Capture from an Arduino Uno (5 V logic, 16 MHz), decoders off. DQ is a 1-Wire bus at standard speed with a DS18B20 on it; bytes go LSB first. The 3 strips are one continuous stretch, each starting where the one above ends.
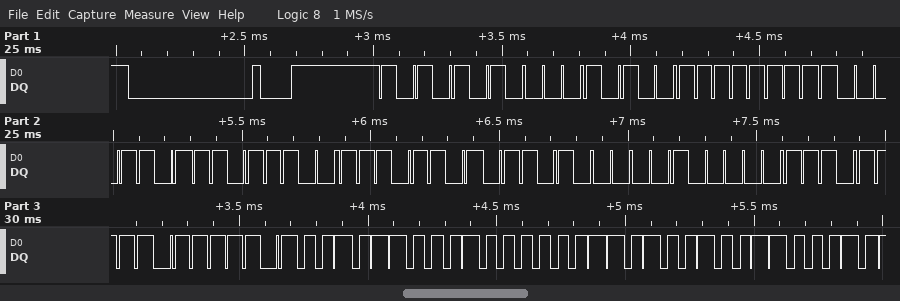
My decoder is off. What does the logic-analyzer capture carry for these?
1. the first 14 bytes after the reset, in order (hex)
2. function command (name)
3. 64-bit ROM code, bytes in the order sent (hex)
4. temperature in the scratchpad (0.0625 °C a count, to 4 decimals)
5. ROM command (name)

55 28 FF B1 3B B7 16 04 F7 BE 34 02 4B 46
Read Scratchpad
28 FF B1 3B B7 16 04 F7
35.2500 °C
Match ROM
